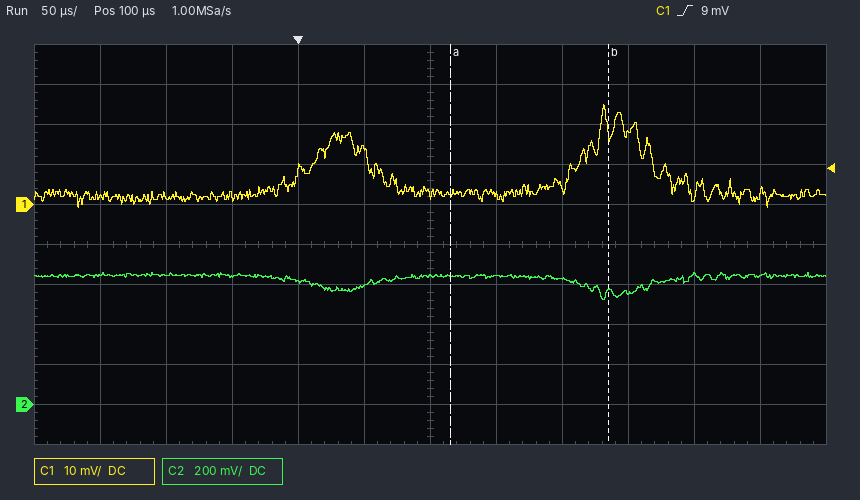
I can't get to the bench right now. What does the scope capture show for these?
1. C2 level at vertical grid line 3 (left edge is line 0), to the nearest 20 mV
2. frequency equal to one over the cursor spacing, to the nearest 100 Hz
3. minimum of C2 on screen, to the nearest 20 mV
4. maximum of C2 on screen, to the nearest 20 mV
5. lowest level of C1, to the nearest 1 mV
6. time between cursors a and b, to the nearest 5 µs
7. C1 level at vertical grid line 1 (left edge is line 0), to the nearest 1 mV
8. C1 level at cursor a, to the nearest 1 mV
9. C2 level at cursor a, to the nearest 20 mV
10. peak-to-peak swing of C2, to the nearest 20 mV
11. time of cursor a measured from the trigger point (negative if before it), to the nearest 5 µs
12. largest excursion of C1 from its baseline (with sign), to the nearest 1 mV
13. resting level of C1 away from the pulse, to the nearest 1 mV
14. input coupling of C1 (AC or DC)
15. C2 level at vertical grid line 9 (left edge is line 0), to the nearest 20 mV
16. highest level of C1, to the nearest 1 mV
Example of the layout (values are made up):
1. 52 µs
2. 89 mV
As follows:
1. 640 mV
2. 8.3 kHz
3. 520 mV
4. 660 mV
5. -1 mV
6. 120 µs
7. 2 mV
8. 3 mV
9. 640 mV
10. 140 mV
11. +115 µs
12. +22 mV
13. 3 mV
14. DC
15. 560 mV
16. 25 mV
